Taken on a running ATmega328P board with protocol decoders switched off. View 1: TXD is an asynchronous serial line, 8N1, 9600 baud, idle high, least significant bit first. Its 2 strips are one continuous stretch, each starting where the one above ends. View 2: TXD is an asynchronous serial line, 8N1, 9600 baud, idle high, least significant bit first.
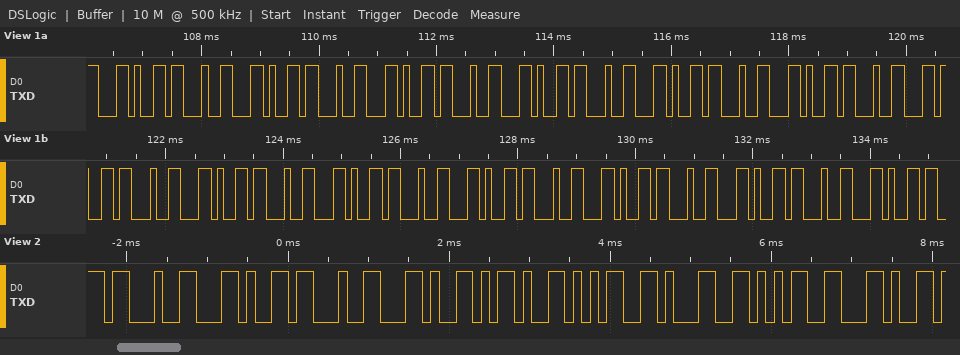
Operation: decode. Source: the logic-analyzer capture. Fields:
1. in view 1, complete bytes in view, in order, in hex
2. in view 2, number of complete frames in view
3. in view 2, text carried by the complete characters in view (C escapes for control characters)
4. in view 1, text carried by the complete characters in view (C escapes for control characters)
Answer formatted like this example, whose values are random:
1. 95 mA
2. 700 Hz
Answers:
1. 2C 23 2C 23 2C 23 2C 23 2C 23 2C 23 2C 23 2C 23 2C 23 2C 23 2C 23 2C 23 2C
2. 9
3. "#,#,-515,"
4. ",#,#,#,#,#,#,#,#,#,#,#,#,"
